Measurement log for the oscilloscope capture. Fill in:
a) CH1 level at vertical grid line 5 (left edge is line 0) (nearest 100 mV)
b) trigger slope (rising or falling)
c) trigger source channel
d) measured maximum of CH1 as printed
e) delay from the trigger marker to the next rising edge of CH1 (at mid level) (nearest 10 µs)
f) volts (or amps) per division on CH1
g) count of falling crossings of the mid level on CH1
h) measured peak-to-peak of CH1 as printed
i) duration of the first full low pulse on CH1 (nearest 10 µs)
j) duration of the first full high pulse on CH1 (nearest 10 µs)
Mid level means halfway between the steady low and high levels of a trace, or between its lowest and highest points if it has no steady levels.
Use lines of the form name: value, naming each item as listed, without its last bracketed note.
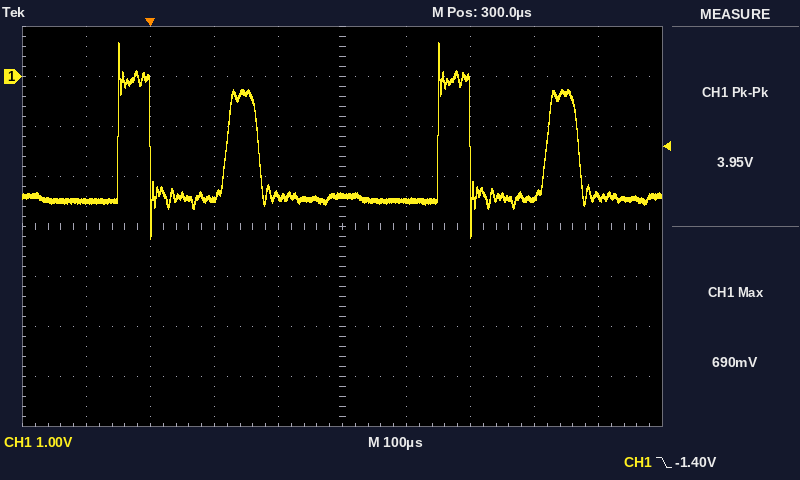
CH1 level at vertical grid line 5 (left edge is line 0): -2.4 V
trigger slope: falling
trigger source channel: CH1
measured maximum of CH1 as printed: 690 mV
delay from the trigger marker to the next rising edge of CH1 (at mid level): 120 µs
volts (or amps) per division on CH1: 1 V
count of falling crossings of the mid level on CH1: 4
measured peak-to-peak of CH1 as printed: 3.95 V
duration of the first full low pulse on CH1: 120 µs
duration of the first full high pulse on CH1: 50 µs
